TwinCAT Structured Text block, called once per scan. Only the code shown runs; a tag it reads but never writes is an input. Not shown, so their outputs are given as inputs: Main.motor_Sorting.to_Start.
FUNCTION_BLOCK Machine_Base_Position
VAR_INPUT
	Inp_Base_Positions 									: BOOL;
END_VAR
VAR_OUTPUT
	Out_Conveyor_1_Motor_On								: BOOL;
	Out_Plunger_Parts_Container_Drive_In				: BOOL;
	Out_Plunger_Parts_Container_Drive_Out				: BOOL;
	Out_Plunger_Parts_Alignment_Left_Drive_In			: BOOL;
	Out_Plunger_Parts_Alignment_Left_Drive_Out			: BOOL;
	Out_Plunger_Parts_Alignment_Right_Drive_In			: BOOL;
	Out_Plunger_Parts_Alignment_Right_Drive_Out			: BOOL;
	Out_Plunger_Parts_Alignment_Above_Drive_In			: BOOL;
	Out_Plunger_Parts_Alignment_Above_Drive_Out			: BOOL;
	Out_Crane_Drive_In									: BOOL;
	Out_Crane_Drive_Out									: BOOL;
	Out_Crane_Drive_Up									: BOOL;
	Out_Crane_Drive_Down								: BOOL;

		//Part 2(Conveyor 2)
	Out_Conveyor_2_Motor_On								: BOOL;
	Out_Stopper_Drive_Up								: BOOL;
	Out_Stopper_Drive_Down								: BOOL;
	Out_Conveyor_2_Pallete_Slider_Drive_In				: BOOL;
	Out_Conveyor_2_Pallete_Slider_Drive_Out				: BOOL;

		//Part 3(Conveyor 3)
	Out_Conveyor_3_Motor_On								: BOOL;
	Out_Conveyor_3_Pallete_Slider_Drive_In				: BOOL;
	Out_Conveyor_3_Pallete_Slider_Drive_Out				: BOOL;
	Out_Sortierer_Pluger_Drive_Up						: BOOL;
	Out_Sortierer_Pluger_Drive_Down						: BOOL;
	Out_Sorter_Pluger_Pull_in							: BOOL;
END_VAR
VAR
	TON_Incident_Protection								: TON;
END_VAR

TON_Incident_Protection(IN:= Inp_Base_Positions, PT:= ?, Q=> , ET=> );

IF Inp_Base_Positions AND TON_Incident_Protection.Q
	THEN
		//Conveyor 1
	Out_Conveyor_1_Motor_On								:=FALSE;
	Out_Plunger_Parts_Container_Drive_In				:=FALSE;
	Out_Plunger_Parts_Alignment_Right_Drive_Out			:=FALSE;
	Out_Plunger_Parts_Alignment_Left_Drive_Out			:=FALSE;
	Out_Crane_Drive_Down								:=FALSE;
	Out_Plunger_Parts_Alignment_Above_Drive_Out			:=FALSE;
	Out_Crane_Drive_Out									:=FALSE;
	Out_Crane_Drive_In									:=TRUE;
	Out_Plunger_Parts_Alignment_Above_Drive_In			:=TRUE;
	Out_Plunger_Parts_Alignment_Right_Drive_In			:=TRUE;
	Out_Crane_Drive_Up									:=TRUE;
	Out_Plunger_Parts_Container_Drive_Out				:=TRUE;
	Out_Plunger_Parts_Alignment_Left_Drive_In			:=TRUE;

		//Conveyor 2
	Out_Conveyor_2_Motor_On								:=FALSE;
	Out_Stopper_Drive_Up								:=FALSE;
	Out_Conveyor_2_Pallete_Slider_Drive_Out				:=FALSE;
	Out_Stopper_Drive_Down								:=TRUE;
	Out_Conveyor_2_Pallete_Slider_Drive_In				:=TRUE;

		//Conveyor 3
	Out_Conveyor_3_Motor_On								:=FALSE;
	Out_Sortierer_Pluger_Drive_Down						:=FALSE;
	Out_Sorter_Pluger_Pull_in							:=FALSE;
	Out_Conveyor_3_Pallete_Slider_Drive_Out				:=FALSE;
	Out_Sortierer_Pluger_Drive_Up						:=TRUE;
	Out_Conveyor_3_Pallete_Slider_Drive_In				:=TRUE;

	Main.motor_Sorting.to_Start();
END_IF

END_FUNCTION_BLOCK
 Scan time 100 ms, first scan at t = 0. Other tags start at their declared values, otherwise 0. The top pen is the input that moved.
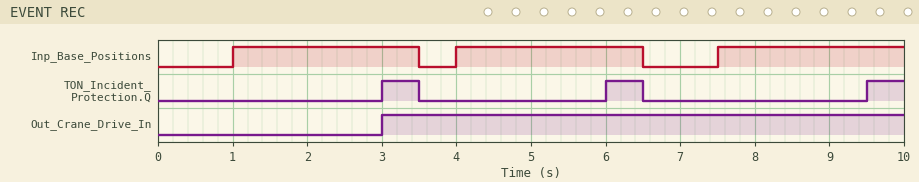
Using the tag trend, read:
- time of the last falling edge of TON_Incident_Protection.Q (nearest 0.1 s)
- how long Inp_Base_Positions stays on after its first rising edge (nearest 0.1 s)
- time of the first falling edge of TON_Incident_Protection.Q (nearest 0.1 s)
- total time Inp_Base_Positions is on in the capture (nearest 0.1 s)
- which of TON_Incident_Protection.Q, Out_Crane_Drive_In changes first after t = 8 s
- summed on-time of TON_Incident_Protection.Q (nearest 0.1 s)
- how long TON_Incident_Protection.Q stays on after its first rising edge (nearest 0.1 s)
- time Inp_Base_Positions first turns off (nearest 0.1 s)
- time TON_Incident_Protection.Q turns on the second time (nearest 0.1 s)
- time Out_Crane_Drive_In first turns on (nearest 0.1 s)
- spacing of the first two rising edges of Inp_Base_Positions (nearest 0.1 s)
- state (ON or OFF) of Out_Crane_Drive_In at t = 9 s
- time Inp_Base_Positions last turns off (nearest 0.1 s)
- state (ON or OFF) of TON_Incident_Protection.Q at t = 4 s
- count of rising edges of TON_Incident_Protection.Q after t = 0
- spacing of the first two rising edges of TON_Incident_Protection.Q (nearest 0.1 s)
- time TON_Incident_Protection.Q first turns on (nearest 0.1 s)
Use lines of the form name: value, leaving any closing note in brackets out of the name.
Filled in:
time of the last falling edge of TON_Incident_Protection.Q: 6.5 s
how long Inp_Base_Positions stays on after its first rising edge: 2.5 s
time of the first falling edge of TON_Incident_Protection.Q: 3.5 s
total time Inp_Base_Positions is on in the capture: 7.5 s
which of TON_Incident_Protection.Q, Out_Crane_Drive_In changes first after t = 8 s: TON_Incident_Protection.Q
summed on-time of TON_Incident_Protection.Q: 1.5 s
how long TON_Incident_Protection.Q stays on after its first rising edge: 0.5 s
time Inp_Base_Positions first turns off: 3.5 s
time TON_Incident_Protection.Q turns on the second time: 6.0 s
time Out_Crane_Drive_In first turns on: 3.0 s
spacing of the first two rising edges of Inp_Base_Positions: 3.0 s
state (ON or OFF) of Out_Crane_Drive_In at t = 9 s: ON
time Inp_Base_Positions last turns off: 6.5 s
state (ON or OFF) of TON_Incident_Protection.Q at t = 4 s: OFF
count of rising edges of TON_Incident_Protection.Q after t = 0: 3
spacing of the first two rising edges of TON_Incident_Protection.Q: 3.0 s
time TON_Incident_Protection.Q first turns on: 3.0 s
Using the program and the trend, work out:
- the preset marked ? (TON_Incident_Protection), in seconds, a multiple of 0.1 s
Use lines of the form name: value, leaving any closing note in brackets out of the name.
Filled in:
the preset marked ? (TON_Incident_Protection), in seconds, a multiple of 0.1 s: 2.0 s
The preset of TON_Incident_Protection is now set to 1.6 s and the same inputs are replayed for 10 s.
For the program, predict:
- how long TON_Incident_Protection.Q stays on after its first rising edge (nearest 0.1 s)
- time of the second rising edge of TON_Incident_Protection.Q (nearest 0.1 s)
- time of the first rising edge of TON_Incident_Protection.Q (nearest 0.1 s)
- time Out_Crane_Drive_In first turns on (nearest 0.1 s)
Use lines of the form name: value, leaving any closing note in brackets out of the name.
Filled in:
how long TON_Incident_Protection.Q stays on after its first rising edge: 0.9 s
time of the second rising edge of TON_Incident_Protection.Q: 5.6 s
time of the first rising edge of TON_Incident_Protection.Q: 2.6 s
time Out_Crane_Drive_In first turns on: 2.6 s
